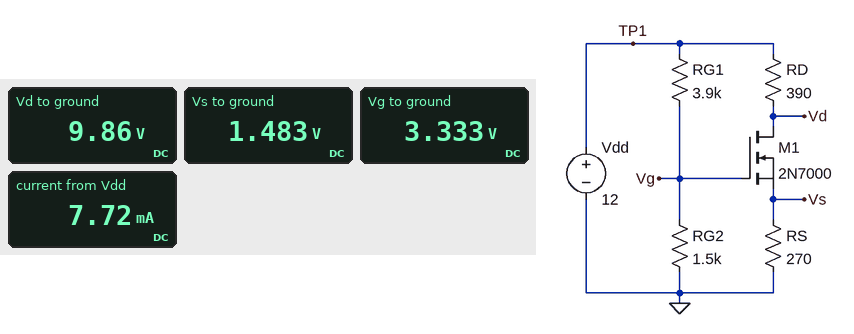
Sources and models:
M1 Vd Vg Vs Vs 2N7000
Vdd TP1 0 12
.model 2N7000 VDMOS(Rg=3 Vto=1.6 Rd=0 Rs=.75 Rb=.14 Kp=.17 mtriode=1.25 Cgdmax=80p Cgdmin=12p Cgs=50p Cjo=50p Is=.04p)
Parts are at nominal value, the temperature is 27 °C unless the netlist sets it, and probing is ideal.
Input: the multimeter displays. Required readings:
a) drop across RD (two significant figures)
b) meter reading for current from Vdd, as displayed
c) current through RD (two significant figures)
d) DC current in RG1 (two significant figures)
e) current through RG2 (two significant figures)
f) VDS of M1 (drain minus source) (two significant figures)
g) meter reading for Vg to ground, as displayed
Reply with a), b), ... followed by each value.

a) 2.1 V
b) 7.72 mA
c) 5.5 mA
d) 2.2 mA
e) 2.2 mA
f) 8.4 V
g) 3.333 V
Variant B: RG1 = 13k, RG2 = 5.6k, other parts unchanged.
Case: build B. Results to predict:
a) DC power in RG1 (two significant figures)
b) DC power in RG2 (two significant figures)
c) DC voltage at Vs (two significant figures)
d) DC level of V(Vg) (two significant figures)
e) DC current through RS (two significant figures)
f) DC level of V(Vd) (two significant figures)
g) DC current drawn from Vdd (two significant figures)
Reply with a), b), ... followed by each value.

a) 5.4 mW
b) 2.3 mW
c) 1.7 V
d) 3.6 V
e) 6.4 mA
f) 9.5 V
g) 7.1 mA
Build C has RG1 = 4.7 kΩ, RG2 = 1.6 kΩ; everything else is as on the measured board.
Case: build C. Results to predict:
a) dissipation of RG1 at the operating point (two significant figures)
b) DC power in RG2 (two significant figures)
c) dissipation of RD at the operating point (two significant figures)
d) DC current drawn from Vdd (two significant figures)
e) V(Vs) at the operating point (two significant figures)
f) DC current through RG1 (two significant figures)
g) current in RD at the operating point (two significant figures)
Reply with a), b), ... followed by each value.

a) 17 mW
b) 5.8 mW
c) 8.0 mW
d) 6.4 mA
e) 1.2 V
f) 1.9 mA
g) 4.5 mA
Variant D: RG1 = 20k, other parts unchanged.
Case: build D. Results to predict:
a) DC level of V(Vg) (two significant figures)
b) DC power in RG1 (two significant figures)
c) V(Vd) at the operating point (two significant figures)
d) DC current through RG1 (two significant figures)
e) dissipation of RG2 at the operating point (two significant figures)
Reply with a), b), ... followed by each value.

a) 840 mV
b) 6.2 mW
c) 12 V
d) 560 µA
e) 470 µW
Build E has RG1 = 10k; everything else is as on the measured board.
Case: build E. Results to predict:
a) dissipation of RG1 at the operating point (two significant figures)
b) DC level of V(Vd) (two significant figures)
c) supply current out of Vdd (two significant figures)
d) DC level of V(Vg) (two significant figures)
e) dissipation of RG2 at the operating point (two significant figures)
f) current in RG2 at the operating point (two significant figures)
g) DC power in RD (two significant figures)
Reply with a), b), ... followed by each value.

a) 11 mW
b) 12 V
c) 1.2 mA
d) 1.6 V
e) 1.6 mW
f) 1.0 mA
g) 7.1 µW
